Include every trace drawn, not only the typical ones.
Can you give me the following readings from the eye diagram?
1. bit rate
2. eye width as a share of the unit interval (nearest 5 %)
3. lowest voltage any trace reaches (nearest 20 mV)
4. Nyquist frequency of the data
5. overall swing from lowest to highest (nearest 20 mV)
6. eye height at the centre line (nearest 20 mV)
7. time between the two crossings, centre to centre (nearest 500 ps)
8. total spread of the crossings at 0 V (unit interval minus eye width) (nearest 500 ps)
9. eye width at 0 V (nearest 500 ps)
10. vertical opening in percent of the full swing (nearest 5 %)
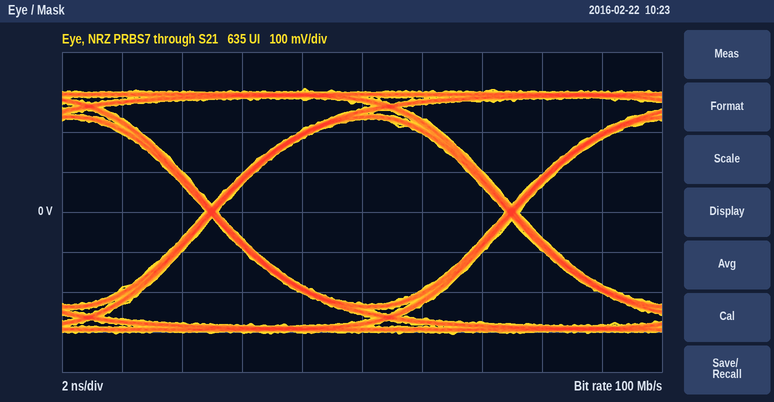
100 Mb/s
95 %
-300 mV
50 MHz
620 mV
460 mV
10.0 ns
500 ps
9.5 ns
75 %
